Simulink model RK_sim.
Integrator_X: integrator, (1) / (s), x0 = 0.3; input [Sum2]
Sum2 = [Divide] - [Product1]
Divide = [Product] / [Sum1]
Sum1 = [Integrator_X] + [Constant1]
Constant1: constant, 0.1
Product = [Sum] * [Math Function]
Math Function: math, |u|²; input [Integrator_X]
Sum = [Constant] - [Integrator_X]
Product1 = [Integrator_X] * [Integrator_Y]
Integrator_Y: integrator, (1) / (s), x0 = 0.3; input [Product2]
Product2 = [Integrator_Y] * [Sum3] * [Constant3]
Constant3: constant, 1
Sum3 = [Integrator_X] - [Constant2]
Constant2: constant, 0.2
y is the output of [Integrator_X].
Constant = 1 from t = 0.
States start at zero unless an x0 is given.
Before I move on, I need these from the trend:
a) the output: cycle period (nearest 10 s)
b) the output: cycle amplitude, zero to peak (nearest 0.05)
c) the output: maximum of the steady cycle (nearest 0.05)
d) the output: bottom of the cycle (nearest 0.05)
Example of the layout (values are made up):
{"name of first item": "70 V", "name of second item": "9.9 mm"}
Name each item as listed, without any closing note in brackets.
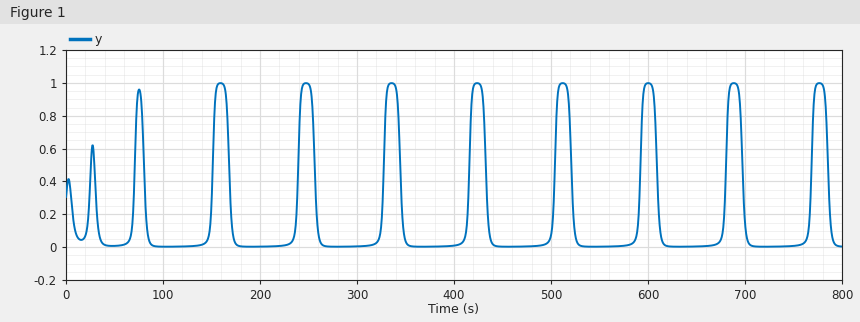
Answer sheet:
{"the output: cycle period": "90 s", "the output: cycle amplitude, zero to peak": "0.50", "the output: maximum of the steady cycle": "1.00", "the output: bottom of the cycle": "0.00"}
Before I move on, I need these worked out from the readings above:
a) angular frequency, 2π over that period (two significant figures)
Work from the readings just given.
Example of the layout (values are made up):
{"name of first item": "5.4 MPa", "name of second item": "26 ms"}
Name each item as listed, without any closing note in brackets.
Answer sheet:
{"angular frequency, 2π over that period": "0.070 rad/s"}
